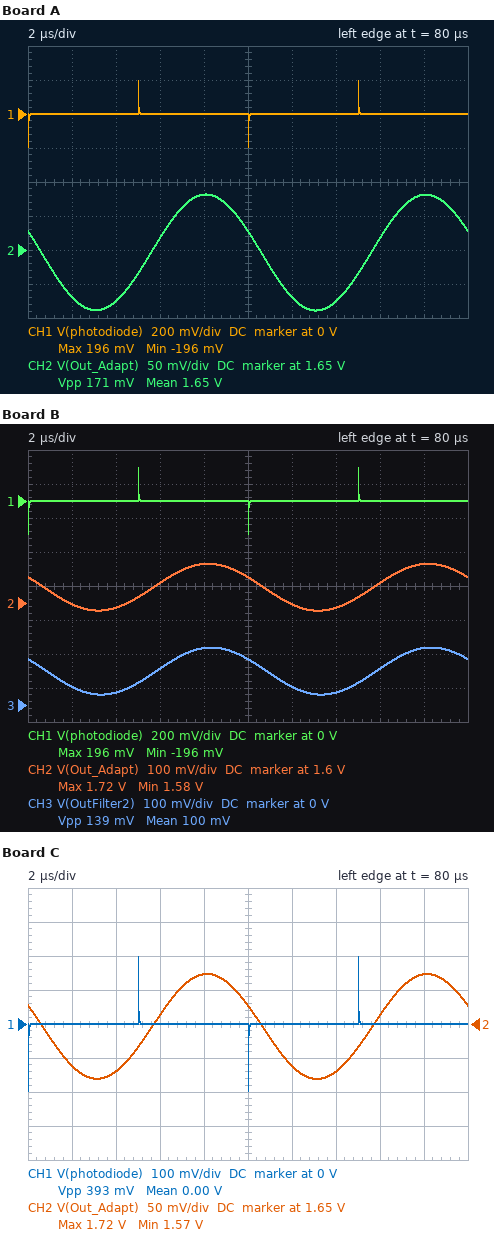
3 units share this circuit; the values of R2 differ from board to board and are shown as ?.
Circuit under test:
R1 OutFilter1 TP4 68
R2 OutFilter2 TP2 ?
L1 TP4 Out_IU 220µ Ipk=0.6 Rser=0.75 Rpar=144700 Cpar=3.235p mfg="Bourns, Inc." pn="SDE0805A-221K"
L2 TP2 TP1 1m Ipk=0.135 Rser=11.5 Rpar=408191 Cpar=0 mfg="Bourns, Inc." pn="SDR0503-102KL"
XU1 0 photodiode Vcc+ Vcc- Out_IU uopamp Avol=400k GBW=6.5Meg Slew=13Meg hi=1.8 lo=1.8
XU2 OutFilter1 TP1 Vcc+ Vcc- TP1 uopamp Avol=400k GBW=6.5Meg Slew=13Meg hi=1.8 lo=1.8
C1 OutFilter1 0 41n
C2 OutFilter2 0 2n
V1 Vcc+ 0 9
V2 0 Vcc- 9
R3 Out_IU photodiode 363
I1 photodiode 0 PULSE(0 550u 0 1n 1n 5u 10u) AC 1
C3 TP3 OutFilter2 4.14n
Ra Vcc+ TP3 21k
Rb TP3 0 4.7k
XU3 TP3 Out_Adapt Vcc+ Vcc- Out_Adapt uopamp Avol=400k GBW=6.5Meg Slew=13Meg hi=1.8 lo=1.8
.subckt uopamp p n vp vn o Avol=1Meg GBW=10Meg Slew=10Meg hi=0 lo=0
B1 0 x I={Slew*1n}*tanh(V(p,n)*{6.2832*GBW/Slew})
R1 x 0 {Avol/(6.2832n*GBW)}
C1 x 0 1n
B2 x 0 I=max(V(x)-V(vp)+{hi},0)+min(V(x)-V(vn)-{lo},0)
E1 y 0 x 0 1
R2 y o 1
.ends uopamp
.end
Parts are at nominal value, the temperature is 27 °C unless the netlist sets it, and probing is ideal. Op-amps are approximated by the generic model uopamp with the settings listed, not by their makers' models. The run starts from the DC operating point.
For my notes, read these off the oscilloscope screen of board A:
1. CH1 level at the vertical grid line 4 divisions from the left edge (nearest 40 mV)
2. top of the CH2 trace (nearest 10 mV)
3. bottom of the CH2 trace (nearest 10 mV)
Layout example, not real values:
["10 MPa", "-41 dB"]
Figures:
["0 V", "1.73 V", "1.56 V"]
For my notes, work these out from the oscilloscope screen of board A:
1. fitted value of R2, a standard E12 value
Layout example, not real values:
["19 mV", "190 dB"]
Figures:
["180 Ω"]
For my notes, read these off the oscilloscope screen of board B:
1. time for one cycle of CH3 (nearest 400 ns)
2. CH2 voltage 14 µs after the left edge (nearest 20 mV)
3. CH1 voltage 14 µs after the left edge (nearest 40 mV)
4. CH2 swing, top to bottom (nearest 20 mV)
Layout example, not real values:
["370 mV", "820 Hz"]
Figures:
["10.0 µs", "1.58 V", "0 V", "140 mV"]
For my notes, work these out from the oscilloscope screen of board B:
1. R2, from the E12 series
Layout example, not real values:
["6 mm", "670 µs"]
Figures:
["270 Ω"]
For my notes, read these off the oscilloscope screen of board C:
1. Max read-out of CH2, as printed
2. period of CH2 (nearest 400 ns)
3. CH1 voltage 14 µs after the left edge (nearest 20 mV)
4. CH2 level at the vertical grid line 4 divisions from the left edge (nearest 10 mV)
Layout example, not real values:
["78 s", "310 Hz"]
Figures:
["1.72 V", "10.0 µs", "0 V", "1.72 V"]
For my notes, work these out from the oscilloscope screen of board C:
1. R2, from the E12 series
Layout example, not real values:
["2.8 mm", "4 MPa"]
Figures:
["220 Ω"]
